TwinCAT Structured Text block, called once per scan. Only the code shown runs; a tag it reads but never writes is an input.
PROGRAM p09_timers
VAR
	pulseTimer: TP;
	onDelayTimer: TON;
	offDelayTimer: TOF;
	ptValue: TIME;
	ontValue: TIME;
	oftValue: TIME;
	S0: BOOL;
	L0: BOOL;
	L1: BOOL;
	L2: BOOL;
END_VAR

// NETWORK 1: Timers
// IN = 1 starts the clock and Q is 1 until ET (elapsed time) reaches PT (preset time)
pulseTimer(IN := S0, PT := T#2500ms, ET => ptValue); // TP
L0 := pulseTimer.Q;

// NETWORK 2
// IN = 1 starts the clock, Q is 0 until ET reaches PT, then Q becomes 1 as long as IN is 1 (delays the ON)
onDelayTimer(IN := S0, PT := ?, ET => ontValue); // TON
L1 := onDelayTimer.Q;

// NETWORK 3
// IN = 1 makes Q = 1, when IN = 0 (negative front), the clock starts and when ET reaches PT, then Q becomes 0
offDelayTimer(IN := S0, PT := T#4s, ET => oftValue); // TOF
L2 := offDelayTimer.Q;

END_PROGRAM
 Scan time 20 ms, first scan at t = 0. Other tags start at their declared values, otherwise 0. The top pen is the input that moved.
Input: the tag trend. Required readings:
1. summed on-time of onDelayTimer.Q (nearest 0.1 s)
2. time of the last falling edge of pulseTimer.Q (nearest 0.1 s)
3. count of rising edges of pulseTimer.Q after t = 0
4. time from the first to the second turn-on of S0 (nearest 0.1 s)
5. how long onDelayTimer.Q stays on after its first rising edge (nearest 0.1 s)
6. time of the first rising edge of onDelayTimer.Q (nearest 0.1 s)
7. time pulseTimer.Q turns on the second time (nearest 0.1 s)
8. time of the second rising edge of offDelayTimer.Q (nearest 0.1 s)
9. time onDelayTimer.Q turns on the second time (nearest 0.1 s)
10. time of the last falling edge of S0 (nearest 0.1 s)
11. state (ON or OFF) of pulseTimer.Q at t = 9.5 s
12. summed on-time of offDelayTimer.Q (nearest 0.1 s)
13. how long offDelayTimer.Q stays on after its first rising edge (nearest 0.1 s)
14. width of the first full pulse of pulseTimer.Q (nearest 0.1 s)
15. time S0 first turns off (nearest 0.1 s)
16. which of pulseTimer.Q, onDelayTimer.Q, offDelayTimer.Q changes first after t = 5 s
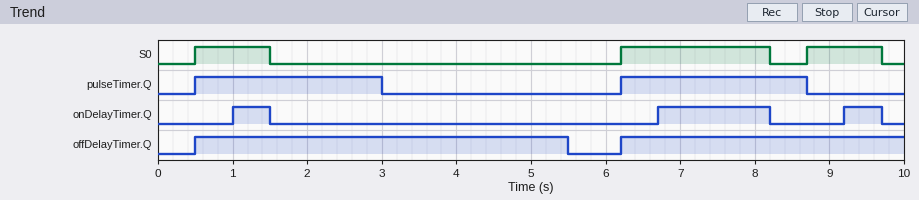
2.5 s
8.7 s
2
5.7 s
0.5 s
1.0 s
6.2 s
6.2 s
6.7 s
9.7 s
OFF
8.8 s
5.0 s
2.5 s
1.5 s
offDelayTimer.Q
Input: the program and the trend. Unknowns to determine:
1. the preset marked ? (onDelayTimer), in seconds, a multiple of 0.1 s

0.5 s
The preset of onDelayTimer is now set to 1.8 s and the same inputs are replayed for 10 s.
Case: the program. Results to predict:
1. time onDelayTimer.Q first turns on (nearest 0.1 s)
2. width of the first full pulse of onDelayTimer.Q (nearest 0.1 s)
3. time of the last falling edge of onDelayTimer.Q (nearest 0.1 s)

8.0 s
0.2 s
8.2 s
